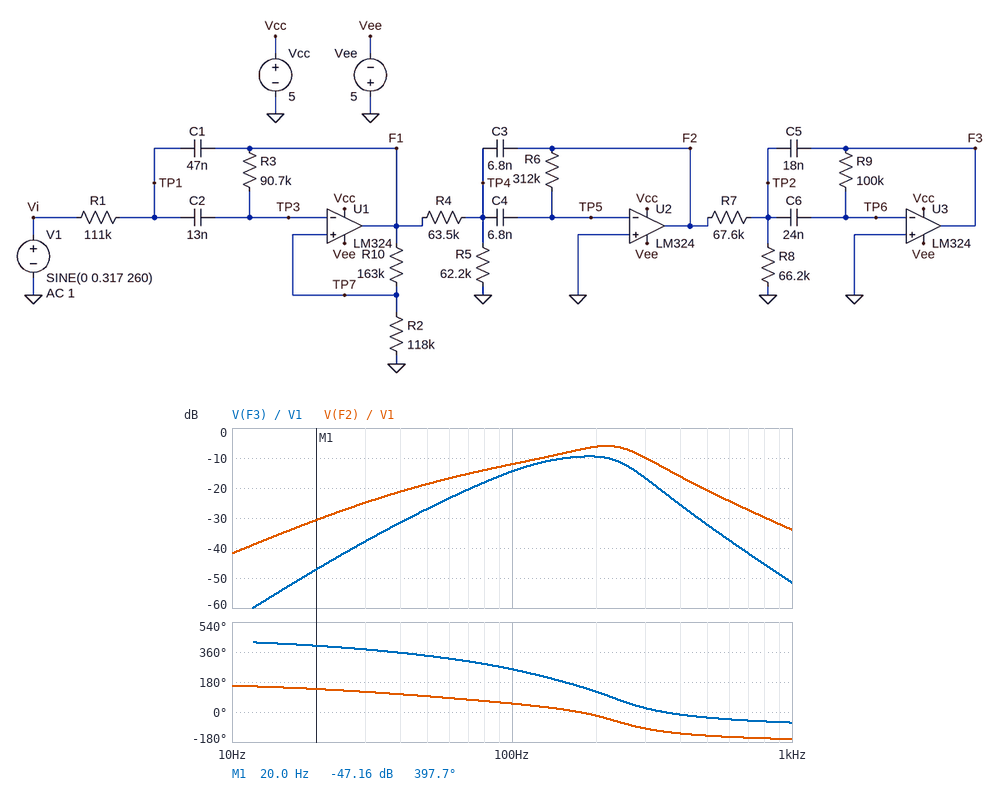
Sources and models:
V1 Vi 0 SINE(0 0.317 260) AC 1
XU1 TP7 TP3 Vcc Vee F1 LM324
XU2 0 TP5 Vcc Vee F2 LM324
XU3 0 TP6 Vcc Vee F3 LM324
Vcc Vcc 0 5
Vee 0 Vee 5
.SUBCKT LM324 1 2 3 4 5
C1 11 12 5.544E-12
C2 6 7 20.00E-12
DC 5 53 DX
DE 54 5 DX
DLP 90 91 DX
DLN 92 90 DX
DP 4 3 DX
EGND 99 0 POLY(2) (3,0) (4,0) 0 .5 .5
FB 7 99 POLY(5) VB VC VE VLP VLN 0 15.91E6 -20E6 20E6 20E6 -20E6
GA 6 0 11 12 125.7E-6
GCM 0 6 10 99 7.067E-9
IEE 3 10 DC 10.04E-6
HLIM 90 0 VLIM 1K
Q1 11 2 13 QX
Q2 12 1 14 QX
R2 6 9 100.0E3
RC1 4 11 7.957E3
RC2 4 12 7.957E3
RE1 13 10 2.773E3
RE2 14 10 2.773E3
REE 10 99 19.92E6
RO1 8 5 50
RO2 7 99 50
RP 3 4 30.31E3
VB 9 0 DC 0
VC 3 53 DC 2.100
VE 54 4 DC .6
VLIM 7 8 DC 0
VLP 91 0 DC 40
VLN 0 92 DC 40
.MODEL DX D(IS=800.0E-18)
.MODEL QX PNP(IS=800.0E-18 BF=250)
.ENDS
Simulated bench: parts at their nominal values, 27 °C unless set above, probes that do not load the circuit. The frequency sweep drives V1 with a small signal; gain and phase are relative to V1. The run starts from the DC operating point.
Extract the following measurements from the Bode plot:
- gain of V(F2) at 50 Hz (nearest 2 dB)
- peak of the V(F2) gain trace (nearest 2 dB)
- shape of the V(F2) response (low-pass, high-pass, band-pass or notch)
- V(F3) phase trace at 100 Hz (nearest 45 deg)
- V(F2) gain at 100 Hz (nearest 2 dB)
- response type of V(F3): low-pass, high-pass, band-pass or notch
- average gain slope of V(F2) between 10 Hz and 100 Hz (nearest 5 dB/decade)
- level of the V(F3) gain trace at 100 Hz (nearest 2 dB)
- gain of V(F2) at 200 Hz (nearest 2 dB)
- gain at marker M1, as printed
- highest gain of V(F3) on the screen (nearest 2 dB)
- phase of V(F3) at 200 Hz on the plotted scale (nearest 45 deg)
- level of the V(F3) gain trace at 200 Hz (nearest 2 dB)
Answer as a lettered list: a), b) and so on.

a) -18 dB
b) -6 dB
c) band-pass
d) 270 deg
e) -12 dB
f) band-pass
g) 30 dB/decade
h) -14 dB
i) -6 dB
j) -47.16 dB
k) -10 dB
l) 135 deg
m) -10 dB
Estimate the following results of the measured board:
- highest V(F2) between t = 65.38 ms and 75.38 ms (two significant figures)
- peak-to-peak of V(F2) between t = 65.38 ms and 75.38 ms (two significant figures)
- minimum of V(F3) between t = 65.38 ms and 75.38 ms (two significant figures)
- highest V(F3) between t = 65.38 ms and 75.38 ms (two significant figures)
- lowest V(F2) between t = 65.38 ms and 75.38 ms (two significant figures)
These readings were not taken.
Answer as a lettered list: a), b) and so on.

a) 130 mV
b) 270 mV
c) -74 mV
d) 70 mV
e) -140 mV
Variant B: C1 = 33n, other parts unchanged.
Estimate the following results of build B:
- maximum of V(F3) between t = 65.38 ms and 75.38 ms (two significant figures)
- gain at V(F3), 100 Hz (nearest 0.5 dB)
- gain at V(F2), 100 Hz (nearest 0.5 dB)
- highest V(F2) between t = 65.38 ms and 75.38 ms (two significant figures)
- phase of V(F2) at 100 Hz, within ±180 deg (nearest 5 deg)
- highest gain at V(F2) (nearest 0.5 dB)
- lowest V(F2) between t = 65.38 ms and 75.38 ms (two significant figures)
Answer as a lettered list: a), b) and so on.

a) 100 mV
b) -11.5 dB
c) -9.0 dB
d) 190 mV
e) 55 deg
f) -3.0 dB
g) -200 mV
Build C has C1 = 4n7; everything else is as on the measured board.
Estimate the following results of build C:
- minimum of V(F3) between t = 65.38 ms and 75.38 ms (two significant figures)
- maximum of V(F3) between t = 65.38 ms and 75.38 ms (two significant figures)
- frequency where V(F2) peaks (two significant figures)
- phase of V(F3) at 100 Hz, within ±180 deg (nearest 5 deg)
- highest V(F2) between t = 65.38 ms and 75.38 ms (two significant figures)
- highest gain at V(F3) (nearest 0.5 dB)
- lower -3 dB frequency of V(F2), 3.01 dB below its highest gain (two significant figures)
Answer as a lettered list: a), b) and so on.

a) -680 mV
b) 680 mV
c) 230 Hz
d) -35 deg
e) 1.3 V
f) 9.0 dB
g) 170 Hz
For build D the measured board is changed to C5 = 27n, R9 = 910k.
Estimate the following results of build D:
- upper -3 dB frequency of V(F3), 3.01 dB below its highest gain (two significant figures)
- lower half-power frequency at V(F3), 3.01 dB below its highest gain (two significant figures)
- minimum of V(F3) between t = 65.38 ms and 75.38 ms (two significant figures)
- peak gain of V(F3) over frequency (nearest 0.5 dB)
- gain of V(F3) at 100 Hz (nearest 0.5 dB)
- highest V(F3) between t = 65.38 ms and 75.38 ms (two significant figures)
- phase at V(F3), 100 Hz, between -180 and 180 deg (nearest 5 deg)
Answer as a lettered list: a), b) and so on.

a) 52 Hz
b) 32 Hz
c) -65 mV
d) -6.0 dB
e) -12.0 dB
f) 29 mV
g) 150 deg
